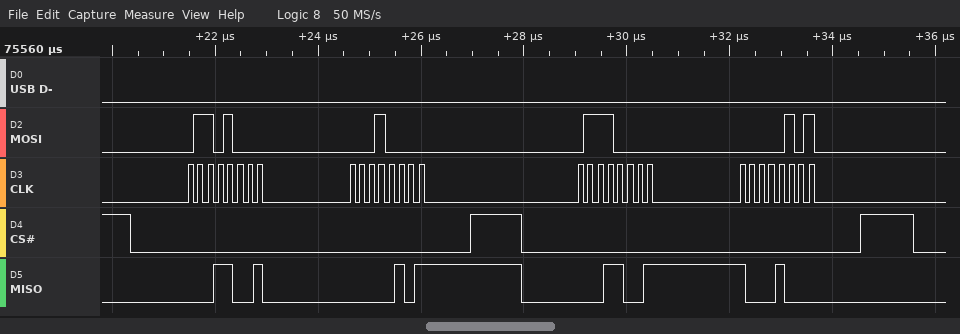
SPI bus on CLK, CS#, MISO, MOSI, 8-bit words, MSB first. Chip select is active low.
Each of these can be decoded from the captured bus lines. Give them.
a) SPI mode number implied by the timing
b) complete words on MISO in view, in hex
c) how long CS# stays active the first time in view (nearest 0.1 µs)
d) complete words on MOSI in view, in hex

0
19, 05, 19, 88
6.6 µs
68, 10, 70, 05
